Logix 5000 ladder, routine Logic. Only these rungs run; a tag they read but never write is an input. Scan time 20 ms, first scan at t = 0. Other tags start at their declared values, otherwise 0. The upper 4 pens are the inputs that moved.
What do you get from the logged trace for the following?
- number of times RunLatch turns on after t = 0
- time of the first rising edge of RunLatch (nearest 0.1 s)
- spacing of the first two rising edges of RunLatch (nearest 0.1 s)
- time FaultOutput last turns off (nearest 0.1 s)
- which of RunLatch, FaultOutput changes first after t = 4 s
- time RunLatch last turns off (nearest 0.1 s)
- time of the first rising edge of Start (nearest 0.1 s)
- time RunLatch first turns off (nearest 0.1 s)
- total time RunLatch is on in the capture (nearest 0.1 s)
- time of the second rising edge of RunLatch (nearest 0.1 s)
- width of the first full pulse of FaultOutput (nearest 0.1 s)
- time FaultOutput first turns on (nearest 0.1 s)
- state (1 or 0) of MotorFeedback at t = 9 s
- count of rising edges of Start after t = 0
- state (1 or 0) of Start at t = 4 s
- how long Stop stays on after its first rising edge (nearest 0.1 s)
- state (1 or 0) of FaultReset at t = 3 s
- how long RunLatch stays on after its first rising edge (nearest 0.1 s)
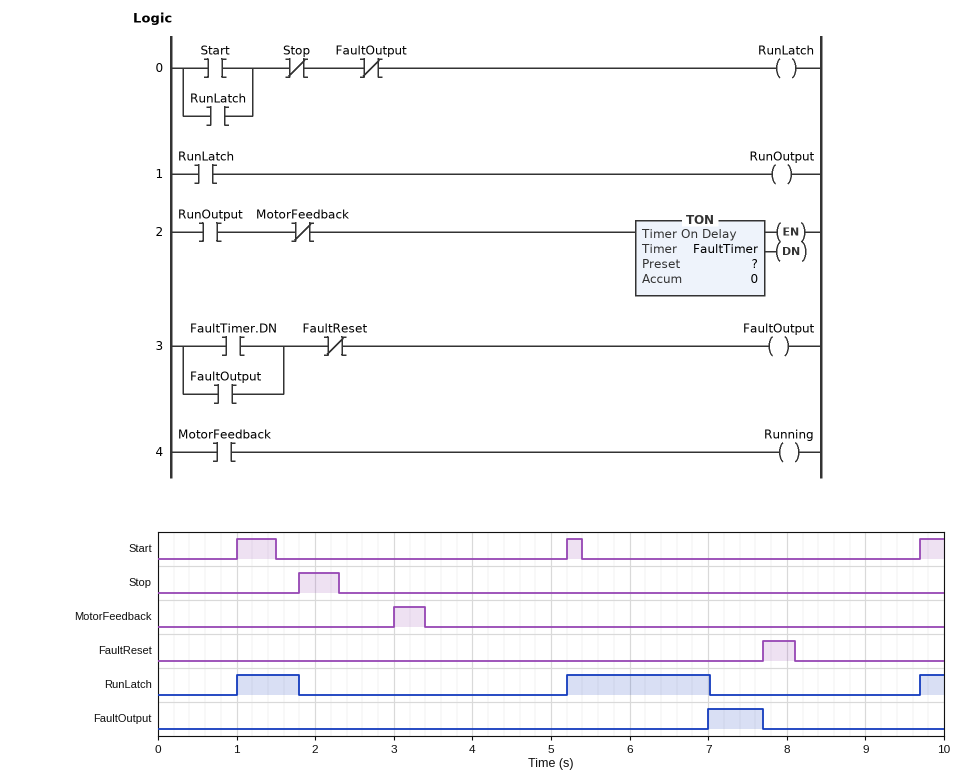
3
1.0 s
4.2 s
7.7 s
RunLatch
7.0 s
1.0 s
1.8 s
2.9 s
5.2 s
0.7 s
7.0 s
0
3
0
0.5 s
0
0.8 s
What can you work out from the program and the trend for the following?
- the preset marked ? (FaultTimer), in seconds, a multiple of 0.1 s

1.8 s
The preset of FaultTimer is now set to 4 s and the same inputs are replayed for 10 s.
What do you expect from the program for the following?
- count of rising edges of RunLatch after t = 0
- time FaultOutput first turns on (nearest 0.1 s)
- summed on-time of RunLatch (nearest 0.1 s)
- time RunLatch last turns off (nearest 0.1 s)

2
9.2 s
4.8 s
9.2 s
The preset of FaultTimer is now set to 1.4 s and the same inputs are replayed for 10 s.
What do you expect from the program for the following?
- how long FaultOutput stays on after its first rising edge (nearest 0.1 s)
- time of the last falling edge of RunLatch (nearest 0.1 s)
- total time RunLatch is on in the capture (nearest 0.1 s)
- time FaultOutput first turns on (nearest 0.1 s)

1.1 s
6.6 s
2.5 s
6.6 s
